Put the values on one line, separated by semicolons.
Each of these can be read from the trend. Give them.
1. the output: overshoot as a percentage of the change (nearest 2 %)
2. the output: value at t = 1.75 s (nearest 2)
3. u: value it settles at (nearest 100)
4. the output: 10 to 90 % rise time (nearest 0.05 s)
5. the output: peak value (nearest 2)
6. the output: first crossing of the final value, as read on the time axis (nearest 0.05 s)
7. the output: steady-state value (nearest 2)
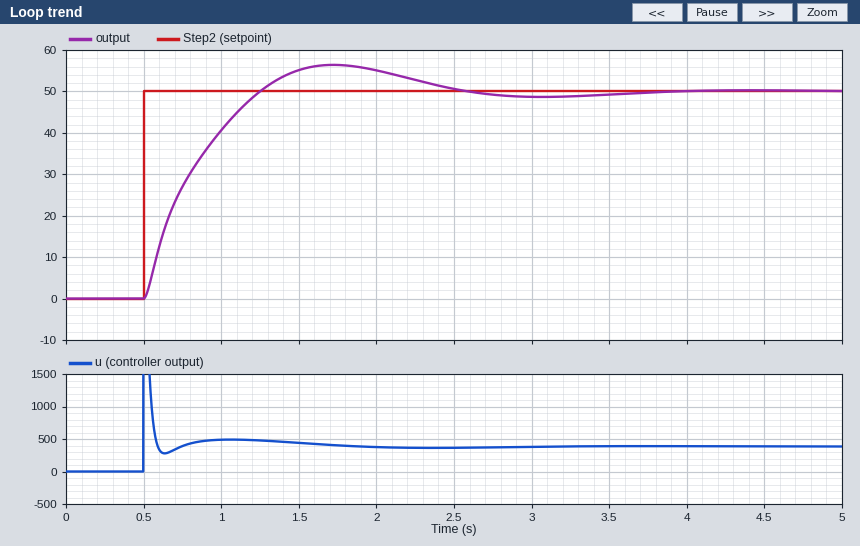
12 %; 56; 400; 0.55 s; 56; 1.25 s; 50
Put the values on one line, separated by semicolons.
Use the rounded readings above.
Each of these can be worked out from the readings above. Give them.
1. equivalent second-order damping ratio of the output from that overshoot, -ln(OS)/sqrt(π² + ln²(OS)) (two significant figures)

0.56
